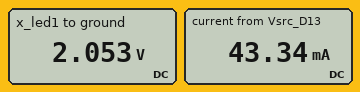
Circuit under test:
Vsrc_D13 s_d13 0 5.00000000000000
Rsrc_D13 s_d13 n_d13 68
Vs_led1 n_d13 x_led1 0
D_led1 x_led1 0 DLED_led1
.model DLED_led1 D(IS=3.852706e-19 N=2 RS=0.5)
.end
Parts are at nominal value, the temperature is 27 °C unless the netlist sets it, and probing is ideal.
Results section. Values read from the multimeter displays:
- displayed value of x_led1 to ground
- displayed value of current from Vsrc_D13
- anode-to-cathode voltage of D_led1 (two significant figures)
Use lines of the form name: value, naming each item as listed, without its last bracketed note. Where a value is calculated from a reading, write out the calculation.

displayed value of x_led1 to ground: 2.053 V
displayed value of current from Vsrc_D13: 43.34 mA
anode-to-cathode voltage of D_led1: 2.053 V = 2.1 V
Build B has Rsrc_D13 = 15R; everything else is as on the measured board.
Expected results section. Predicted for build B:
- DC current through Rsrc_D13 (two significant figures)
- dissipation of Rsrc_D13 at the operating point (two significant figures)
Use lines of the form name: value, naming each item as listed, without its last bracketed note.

DC current through Rsrc_D13: 190 mA
dissipation of Rsrc_D13 at the operating point: 520 mW
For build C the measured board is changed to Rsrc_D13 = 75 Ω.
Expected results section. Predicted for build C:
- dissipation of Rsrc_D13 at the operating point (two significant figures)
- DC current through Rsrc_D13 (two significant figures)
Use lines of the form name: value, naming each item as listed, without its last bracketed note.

dissipation of Rsrc_D13 at the operating point: 120 mW
DC current through Rsrc_D13: 39 mA
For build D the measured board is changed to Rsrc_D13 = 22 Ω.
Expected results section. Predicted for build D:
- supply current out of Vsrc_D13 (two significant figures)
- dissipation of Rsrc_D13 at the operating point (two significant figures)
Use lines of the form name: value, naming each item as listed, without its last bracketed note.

supply current out of Vsrc_D13: 130 mA
dissipation of Rsrc_D13 at the operating point: 370 mW
